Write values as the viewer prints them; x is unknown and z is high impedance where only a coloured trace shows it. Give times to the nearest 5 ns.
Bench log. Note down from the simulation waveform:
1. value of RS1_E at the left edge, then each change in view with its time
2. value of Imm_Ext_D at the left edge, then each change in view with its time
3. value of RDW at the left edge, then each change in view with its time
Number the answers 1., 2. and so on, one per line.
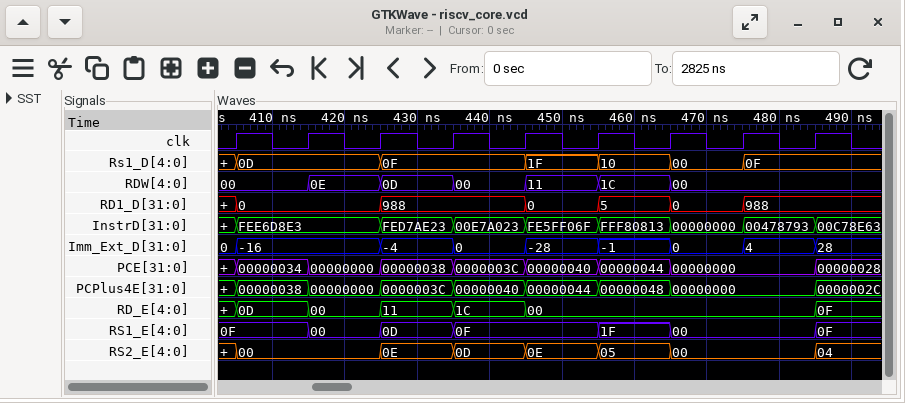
1. 0F, 00 at 415 ns, 0D at 425 ns, 0F at 435 ns, 1F at 455 ns, 00 at 465 ns, 0F at 485 ns
2. 0, -16 at 405 ns, -4 at 425 ns, 0 at 435 ns, -28 at 445 ns, -1 at 455 ns, 0 at 465 ns, 4 at 475 ns, 28 at 485 ns
3. 00, 0E at 415 ns, 0D at 425 ns, 00 at 435 ns, 11 at 445 ns, 1C at 455 ns, 00 at 465 ns
